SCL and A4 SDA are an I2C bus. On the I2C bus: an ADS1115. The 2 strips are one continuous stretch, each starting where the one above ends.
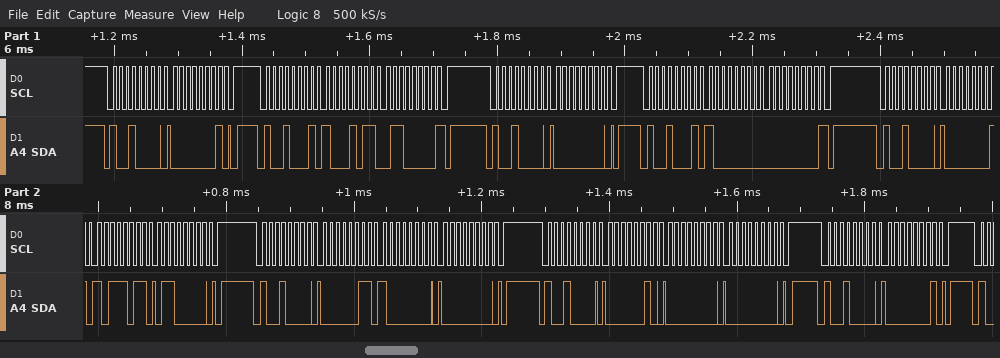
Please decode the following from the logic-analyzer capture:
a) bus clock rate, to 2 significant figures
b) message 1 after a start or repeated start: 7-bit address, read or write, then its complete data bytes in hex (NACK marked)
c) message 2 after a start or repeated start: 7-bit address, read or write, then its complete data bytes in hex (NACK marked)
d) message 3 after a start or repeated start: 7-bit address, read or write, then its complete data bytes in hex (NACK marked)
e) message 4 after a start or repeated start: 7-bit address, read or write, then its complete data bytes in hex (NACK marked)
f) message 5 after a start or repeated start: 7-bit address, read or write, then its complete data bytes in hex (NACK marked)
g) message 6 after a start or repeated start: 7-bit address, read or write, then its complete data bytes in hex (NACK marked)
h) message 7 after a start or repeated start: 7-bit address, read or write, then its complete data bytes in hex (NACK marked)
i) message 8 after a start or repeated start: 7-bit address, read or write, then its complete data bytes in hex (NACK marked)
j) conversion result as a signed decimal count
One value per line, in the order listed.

100 kHz
0x48 write: 01
0x48 read: 8B 60 NACK
0x48 write: 00
0x48 read: 80 00 NACK
0x48 write: 01 BB 60
0x48 write: 03 80 00
0x48 write: 02 00 00
0x48 write: 01
-32768
